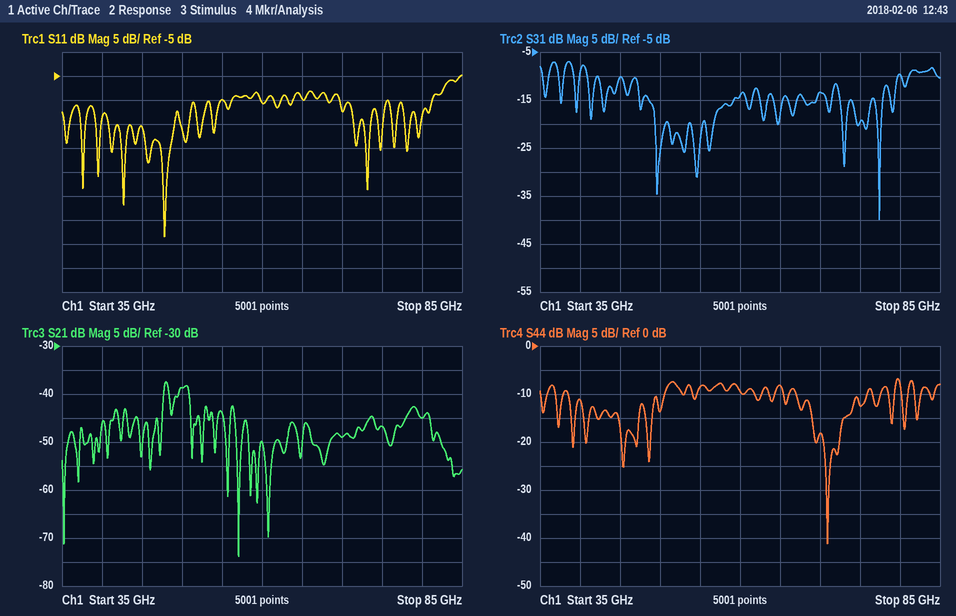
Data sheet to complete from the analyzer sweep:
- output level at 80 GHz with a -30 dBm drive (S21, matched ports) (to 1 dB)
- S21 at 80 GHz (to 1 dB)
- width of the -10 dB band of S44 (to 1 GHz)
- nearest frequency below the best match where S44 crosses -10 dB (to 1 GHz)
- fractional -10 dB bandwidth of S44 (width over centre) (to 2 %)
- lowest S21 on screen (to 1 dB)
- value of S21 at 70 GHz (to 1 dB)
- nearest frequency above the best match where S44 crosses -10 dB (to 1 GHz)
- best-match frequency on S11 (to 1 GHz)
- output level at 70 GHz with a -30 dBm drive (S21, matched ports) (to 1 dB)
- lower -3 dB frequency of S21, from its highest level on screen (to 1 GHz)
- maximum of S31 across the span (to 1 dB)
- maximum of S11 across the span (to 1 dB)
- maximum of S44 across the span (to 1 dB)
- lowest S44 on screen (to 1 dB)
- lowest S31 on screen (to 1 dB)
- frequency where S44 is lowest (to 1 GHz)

-75 dBm
-45 dB
9 GHz
67 GHz
12 %
-74 dB
-49 dB
76 GHz
48 GHz
-79 dBm
48 GHz
-7 dB
-5 dB
-7 dB
-41 dB
-40 dB
71 GHz
